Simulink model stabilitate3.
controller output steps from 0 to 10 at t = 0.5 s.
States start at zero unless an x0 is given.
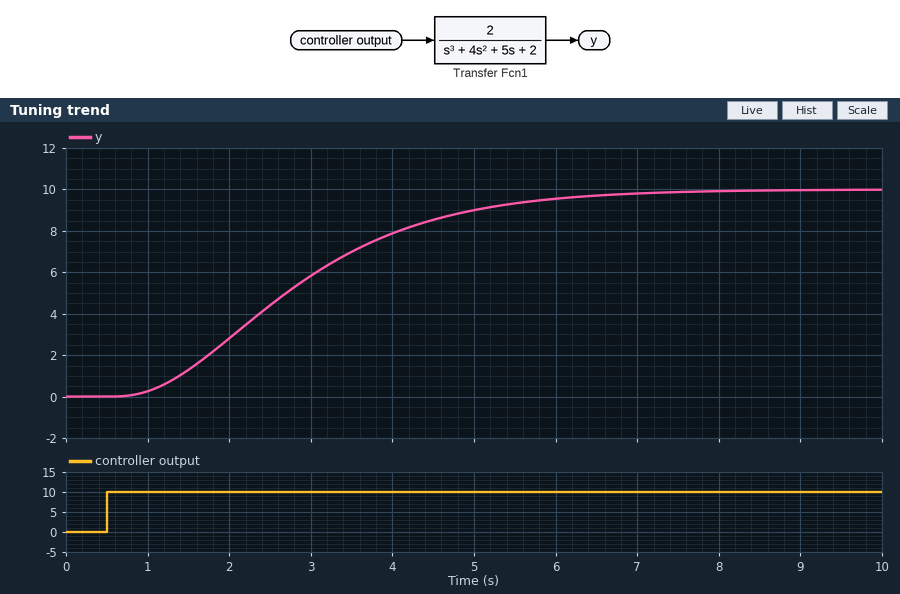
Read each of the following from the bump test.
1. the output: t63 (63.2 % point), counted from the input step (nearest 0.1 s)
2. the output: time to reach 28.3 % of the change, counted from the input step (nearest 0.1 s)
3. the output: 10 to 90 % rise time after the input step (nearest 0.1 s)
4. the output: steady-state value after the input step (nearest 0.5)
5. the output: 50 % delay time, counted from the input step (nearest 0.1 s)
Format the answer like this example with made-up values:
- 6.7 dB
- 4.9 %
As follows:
- 2.7 s
- 1.5 s
- 3.6 s
- 10.0
- 2.2 s
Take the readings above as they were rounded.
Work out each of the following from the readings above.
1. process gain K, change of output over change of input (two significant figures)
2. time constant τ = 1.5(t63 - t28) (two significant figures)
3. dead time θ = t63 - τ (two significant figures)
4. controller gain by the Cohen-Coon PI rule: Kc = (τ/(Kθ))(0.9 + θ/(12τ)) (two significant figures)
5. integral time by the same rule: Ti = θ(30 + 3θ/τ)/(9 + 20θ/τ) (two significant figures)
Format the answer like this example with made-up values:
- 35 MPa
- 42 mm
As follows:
- 1.0
- 1.8 s
- 0.90 s
- 1.9
- 1.5 s
